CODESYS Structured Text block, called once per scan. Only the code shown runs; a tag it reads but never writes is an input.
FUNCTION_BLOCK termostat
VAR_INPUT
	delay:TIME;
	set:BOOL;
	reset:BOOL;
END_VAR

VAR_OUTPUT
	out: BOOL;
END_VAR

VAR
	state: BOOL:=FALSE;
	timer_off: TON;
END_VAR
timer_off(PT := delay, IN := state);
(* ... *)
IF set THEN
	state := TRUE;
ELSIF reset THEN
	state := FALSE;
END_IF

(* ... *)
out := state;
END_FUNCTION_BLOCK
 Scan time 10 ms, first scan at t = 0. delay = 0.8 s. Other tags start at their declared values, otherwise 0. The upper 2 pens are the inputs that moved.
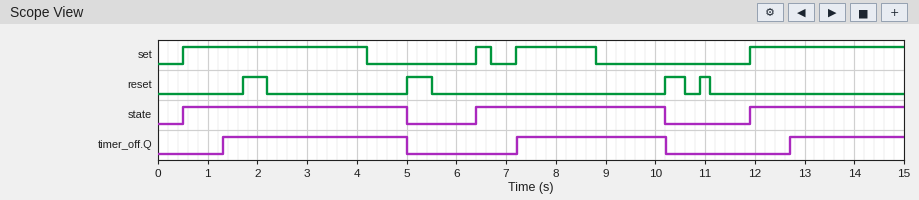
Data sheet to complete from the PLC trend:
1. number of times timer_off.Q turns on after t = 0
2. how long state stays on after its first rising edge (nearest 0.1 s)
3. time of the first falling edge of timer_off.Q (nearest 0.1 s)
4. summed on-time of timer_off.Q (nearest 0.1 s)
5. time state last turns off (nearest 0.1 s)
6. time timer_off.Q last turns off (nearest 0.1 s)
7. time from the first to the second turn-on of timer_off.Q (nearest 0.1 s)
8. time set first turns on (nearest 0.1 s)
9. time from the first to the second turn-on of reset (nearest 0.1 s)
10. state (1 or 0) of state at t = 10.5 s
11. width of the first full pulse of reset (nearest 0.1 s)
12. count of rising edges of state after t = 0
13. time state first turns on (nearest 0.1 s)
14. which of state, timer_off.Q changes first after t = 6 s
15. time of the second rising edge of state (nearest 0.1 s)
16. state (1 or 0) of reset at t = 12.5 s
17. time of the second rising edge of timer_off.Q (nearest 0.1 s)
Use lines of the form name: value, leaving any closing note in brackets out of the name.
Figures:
number of times timer_off.Q turns on after t = 0: 3
how long state stays on after its first rising edge: 4.5 s
time of the first falling edge of timer_off.Q: 5.0 s
summed on-time of timer_off.Q: 9.0 s
time state last turns off: 10.2 s
time timer_off.Q last turns off: 10.2 s
time from the first to the second turn-on of timer_off.Q: 5.9 s
time set first turns on: 0.5 s
time from the first to the second turn-on of reset: 3.3 s
state (1 or 0) of state at t = 10.5 s: 0
width of the first full pulse of reset: 0.5 s
count of rising edges of state after t = 0: 3
time state first turns on: 0.5 s
which of state, timer_off.Q changes first after t = 6 s: state
time of the second rising edge of state: 6.4 s
state (1 or 0) of reset at t = 12.5 s: 0
time of the second rising edge of timer_off.Q: 7.2 s
